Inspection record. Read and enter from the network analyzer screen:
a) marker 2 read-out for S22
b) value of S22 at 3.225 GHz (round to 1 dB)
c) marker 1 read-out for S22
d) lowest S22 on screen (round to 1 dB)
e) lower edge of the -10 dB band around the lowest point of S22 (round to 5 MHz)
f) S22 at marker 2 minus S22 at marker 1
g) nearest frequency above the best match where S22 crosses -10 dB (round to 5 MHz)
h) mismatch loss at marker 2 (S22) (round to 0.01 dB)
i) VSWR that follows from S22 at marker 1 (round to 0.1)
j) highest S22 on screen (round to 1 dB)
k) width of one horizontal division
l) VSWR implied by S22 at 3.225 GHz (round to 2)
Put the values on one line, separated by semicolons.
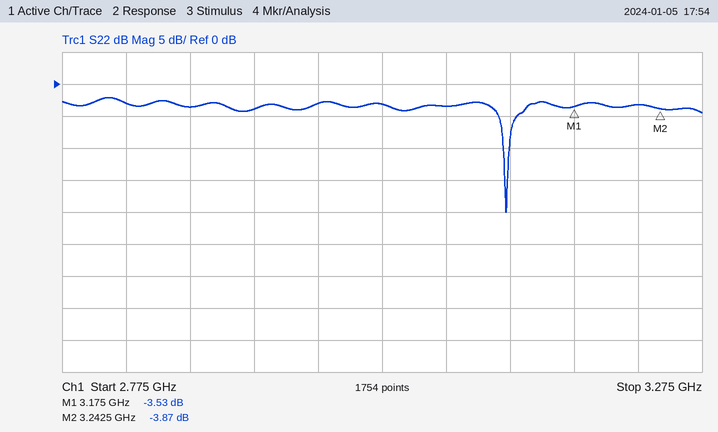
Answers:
-3.87 dB; -3 dB; -3.53 dB; -20 dB; 3.120 GHz; -0.34 dB; 3.125 GHz; 2.29 dB; 5.0; -2 dB; 50 MHz; 6
